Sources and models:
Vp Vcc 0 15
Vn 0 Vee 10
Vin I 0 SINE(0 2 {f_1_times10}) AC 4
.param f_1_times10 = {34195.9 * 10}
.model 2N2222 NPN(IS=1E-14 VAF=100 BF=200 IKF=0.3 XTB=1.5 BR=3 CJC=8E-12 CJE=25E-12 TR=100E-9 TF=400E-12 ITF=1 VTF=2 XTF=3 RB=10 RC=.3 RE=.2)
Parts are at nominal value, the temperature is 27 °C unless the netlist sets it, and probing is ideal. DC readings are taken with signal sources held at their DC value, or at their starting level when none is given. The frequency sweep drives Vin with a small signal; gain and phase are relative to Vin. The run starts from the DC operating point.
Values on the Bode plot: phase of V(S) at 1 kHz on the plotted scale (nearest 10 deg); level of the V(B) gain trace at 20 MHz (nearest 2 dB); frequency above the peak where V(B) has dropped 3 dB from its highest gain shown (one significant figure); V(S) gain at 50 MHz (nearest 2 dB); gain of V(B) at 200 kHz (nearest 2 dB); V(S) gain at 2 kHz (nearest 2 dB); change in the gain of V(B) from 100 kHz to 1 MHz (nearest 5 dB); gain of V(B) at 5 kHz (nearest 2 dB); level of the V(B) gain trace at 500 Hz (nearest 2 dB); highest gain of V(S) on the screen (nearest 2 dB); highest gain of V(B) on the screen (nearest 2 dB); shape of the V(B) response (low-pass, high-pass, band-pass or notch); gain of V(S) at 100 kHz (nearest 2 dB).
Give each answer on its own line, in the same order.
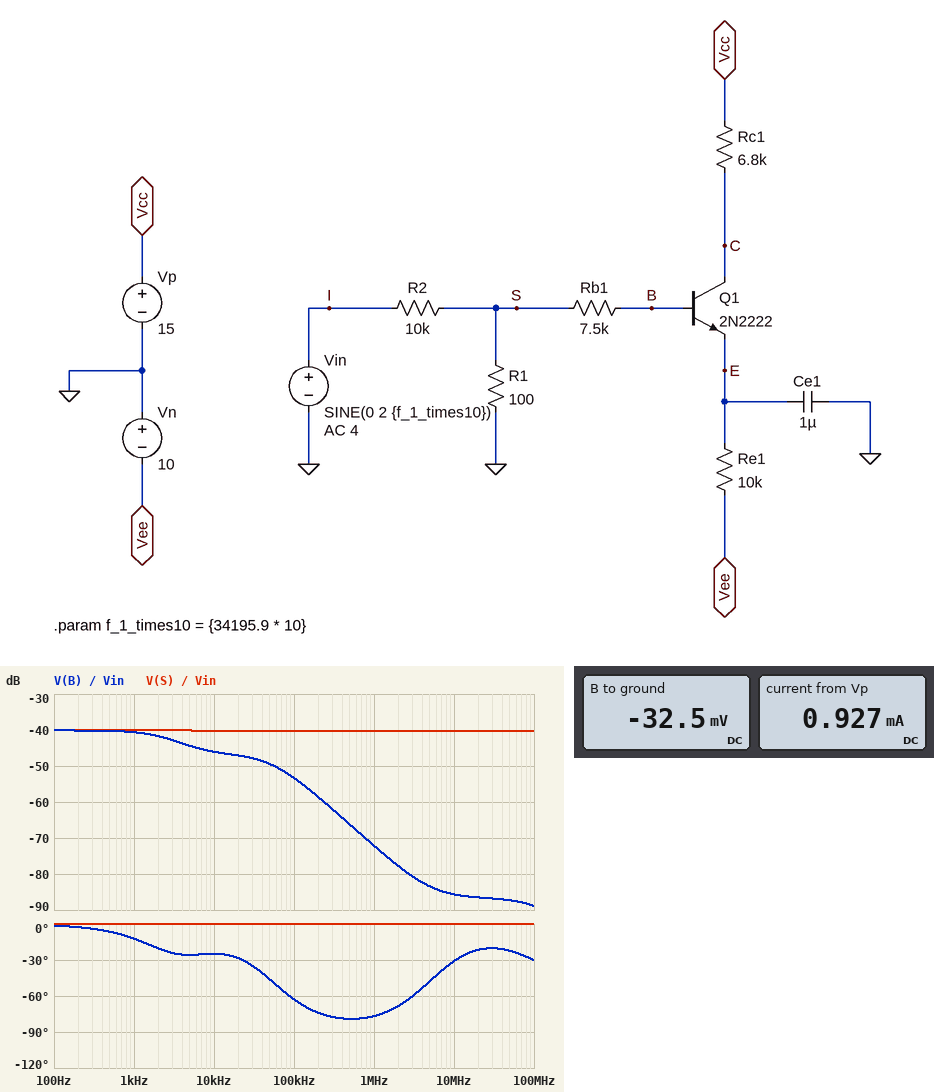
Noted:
0 deg
-86 dB
3 kHz
-40 dB
-58 dB
-40 dB
-20 dB
-44 dB
-40 dB
-40 dB
-40 dB
low-pass
-40 dB
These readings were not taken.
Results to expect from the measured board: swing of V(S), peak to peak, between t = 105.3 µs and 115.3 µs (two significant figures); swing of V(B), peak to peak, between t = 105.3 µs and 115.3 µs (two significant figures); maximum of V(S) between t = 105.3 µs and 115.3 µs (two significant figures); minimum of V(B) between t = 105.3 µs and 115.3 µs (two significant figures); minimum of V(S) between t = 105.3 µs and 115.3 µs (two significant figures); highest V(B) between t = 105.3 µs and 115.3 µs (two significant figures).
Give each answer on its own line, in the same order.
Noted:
39 mV
2.8 mV
19 mV
-34 mV
-20 mV
-31 mV
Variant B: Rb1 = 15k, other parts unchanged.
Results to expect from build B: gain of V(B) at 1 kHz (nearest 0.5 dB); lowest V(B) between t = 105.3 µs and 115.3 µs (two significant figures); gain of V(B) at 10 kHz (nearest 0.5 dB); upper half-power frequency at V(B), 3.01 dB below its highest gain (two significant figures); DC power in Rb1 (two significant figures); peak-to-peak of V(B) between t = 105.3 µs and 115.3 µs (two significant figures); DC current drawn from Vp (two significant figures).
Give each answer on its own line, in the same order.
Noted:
-41.5 dB
-65 mV
-50.0 dB
1.8 kHz
270 nW
1.4 mV
920 µA
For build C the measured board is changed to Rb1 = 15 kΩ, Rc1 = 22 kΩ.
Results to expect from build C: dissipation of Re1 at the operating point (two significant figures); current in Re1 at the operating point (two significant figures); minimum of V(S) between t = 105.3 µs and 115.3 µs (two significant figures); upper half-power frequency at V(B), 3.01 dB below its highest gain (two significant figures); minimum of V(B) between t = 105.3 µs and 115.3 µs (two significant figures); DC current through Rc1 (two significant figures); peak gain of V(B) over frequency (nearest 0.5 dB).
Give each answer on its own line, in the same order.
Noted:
6.9 mW
830 µA
-27 mV
34 Hz
-1.1 V
760 µA
-50.0 dB
